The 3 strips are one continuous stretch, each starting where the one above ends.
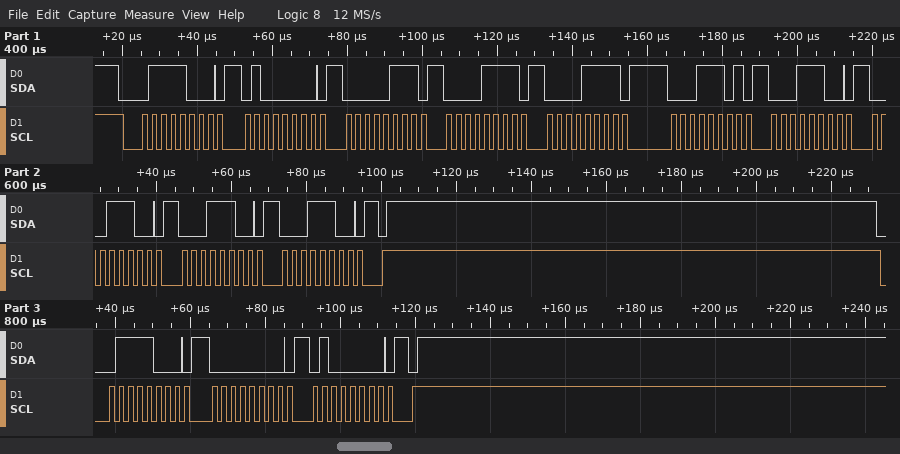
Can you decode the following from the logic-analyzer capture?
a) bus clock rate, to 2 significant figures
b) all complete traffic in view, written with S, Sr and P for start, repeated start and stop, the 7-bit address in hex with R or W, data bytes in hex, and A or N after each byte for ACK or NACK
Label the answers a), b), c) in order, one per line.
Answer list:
a) 400 kHz
b) S 3CW A 40 A 07 A 0F A 0F A 1D A 1C A 1C A 1C A 1C A P S 3CW A 00 A 40 A P
